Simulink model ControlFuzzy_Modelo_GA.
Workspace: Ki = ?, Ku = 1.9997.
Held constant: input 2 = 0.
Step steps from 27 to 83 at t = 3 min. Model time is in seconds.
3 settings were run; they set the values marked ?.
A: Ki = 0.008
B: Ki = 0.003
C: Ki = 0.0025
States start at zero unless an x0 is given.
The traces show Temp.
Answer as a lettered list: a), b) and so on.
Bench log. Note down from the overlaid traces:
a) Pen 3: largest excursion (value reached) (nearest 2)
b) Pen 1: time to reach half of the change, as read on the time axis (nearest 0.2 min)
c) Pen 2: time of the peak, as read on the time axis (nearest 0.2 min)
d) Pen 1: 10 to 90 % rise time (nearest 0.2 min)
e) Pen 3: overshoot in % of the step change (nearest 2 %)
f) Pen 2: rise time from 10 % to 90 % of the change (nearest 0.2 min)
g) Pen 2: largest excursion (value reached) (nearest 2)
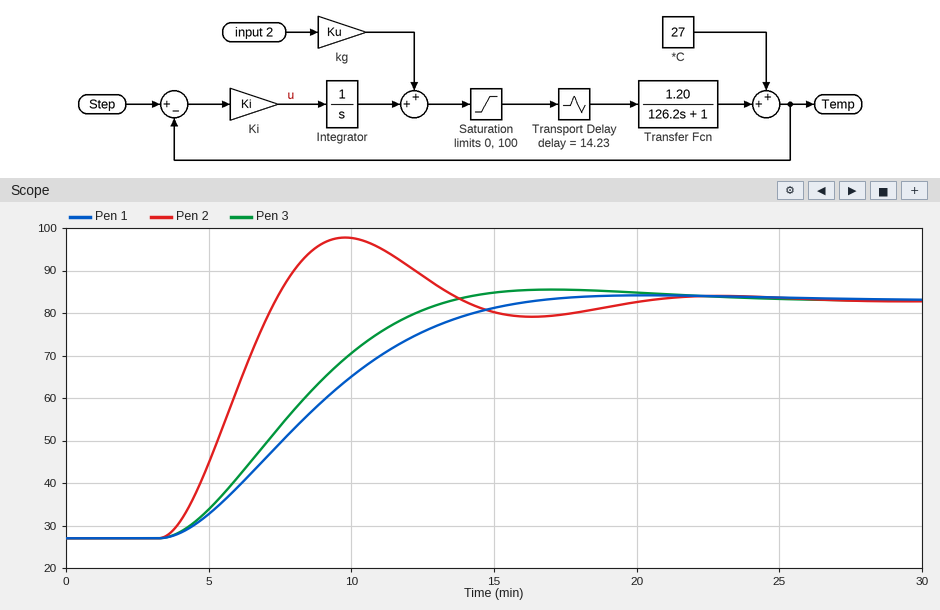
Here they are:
a) 86
b) 8.4 min
c) 9.8 min
d) 8.2 min
e) 4 %
f) 2.8 min
g) 98
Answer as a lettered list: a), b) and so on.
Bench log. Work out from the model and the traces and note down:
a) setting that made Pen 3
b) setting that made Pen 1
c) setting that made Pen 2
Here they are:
a) B
b) C
c) A
